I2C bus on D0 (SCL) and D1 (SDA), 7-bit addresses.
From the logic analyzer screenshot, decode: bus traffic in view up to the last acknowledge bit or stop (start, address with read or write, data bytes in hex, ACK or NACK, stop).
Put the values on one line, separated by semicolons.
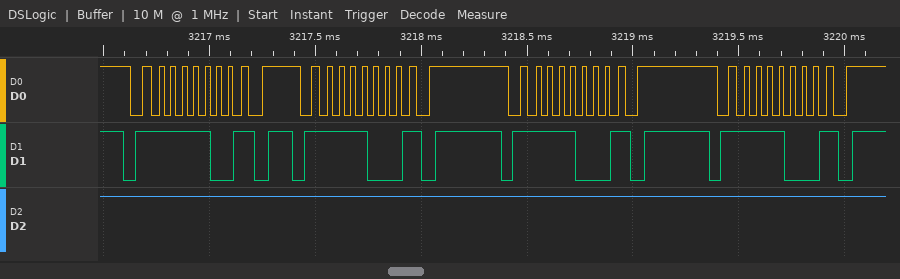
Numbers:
start, address 7E write NACK, stop, start, address 7C write NACK, stop, start, address 7C write NACK, stop, start, address 7C write NACK, stop
